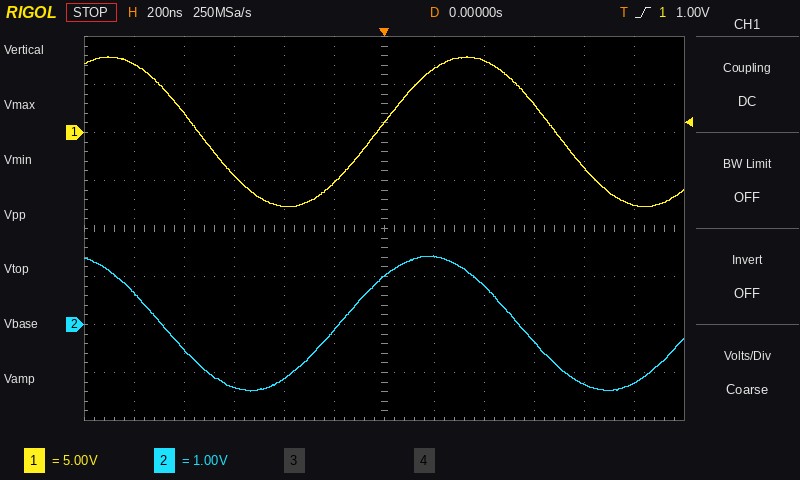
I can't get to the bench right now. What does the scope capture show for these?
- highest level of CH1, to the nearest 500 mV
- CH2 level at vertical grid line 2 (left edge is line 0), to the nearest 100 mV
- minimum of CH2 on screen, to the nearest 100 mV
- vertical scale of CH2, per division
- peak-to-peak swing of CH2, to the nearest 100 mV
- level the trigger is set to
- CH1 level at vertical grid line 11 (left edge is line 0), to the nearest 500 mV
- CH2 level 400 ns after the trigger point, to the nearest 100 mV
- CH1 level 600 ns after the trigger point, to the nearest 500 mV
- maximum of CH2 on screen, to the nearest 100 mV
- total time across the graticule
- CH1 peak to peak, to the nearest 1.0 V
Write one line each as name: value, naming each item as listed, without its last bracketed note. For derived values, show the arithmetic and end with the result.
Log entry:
highest level of CH1, to the nearest 500 mV: 8.0 V
CH2 level at vertical grid line 2 (left edge is line 0), to the nearest 100 mV: -500 mV
minimum of CH2 on screen, to the nearest 100 mV: -1.4 V
vertical scale of CH2, per division: 1 V
peak-to-peak swing of CH2, to the nearest 100 mV: 1.4 V − (-1.4 V) = 2.8 V
level the trigger is set to: 1.00 V
CH1 level at vertical grid line 11 (left edge is line 0), to the nearest 500 mV: -7.5 V
CH2 level 400 ns after the trigger point, to the nearest 100 mV: 800 mV
CH1 level 600 ns after the trigger point, to the nearest 500 mV: 3.0 V
maximum of CH2 on screen, to the nearest 100 mV: 1.4 V
total time across the graticule: 2.4 µs
CH1 peak to peak, to the nearest 1.0 V: 16.0 V
